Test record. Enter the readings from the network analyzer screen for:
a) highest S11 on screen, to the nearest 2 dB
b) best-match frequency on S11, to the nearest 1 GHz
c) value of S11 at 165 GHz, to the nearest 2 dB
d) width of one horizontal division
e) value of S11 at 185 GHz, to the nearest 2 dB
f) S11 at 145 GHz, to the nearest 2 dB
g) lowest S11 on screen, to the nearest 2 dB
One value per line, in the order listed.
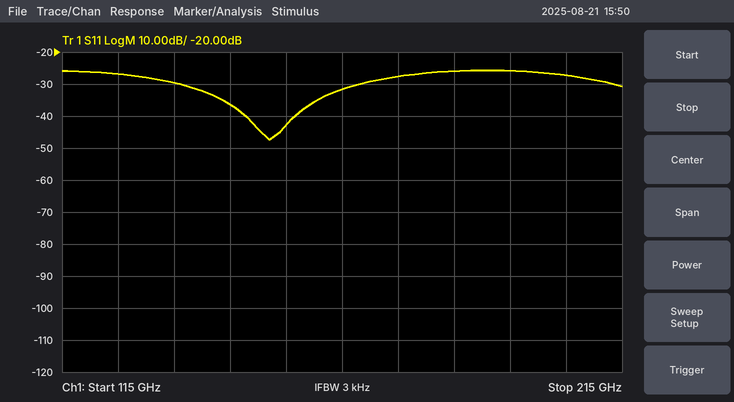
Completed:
-26 dB
152 GHz
-32 dB
10 GHz
-26 dB
-36 dB
-48 dB
